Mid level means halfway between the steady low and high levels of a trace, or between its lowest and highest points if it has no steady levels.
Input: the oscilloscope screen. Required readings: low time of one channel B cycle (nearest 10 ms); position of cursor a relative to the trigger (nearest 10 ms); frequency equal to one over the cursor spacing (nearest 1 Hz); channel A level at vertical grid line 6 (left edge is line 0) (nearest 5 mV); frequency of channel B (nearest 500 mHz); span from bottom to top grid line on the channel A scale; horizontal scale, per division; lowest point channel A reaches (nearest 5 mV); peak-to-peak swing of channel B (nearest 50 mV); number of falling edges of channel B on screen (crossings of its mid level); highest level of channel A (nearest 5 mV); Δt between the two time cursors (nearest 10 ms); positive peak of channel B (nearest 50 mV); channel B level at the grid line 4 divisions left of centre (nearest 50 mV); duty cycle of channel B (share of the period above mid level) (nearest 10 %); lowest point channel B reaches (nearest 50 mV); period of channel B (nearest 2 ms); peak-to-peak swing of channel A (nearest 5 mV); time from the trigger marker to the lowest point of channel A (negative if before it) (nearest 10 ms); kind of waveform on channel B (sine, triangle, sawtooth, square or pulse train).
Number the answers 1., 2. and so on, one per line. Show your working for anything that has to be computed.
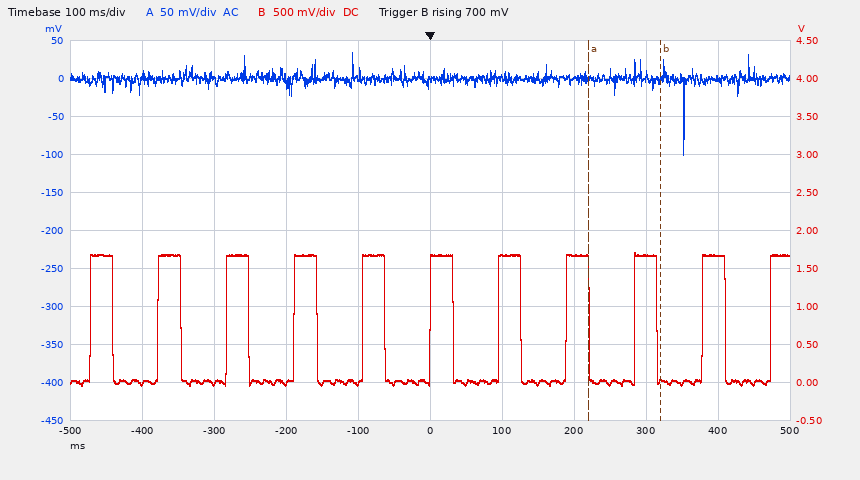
1. 60 ms
2. +220 ms
3. 1 / 100 ms ≈ 10 Hz
4. 0 mV
5. 1 / 94 ms ≈ 10.6 Hz, so 10.5 Hz to the nearest 500 mHz
6. 500 mV
7. 100 ms
8. -100 mV
9. 1.70 V − (-50 mV) = 1.75 V
10. 10
11. 35 mV
12. 100 ms
13. 1.70 V
14. 0 mV
15. 30 %
16. -50 mV
17. 94 ms
18. 35 mV − (-100 mV) = 135 mV
19. +350 ms
20. pulse train
